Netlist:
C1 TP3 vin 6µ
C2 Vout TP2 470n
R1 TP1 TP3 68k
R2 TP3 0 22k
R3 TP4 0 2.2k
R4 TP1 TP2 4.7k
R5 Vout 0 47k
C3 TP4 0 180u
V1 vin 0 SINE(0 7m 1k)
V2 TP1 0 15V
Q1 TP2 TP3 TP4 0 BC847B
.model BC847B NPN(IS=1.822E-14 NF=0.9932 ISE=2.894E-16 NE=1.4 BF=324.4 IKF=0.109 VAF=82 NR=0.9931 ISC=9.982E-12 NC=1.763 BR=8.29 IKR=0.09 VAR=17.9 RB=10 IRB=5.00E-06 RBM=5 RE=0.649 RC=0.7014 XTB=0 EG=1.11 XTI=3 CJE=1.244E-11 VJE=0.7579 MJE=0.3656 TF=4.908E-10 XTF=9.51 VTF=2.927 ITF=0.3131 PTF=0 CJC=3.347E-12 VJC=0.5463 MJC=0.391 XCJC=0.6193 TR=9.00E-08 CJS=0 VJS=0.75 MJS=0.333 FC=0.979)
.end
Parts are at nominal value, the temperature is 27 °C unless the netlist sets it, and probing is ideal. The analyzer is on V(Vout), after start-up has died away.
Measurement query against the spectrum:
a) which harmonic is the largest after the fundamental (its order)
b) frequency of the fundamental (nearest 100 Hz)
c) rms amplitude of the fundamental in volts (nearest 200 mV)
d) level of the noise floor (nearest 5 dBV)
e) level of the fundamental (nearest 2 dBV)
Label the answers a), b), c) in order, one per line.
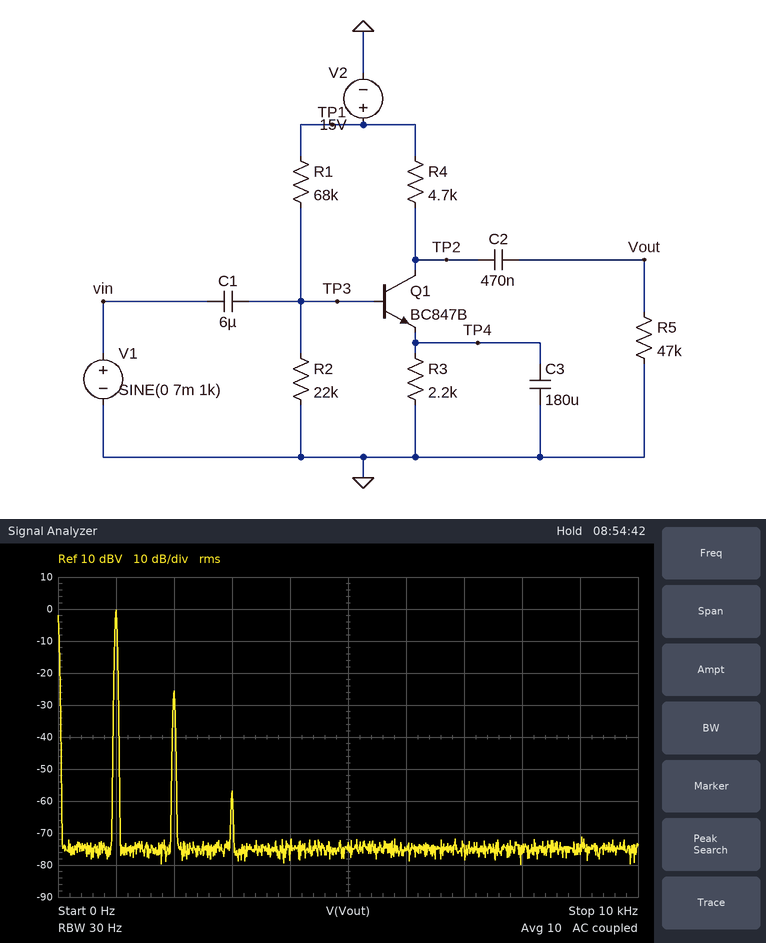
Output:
a) 2
b) 1.0 kHz
c) 1.0 V
d) -75 dBV
e) 0 dBV
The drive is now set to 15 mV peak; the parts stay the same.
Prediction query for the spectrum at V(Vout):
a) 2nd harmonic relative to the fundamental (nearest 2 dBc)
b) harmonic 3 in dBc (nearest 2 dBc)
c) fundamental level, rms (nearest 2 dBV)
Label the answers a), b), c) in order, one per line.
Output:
a) -18 dBc
b) -44 dBc
c) 6 dBV
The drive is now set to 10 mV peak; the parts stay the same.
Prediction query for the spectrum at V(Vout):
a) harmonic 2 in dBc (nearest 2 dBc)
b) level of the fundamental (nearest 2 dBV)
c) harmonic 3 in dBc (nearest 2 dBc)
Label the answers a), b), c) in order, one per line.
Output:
a) -22 dBc
b) 2 dBV
c) -50 dBc
